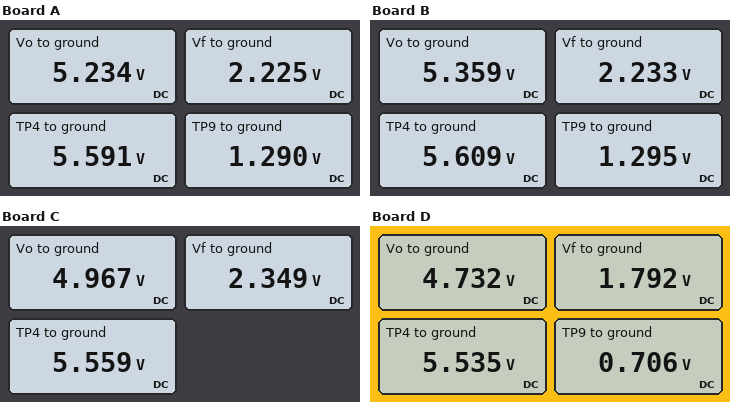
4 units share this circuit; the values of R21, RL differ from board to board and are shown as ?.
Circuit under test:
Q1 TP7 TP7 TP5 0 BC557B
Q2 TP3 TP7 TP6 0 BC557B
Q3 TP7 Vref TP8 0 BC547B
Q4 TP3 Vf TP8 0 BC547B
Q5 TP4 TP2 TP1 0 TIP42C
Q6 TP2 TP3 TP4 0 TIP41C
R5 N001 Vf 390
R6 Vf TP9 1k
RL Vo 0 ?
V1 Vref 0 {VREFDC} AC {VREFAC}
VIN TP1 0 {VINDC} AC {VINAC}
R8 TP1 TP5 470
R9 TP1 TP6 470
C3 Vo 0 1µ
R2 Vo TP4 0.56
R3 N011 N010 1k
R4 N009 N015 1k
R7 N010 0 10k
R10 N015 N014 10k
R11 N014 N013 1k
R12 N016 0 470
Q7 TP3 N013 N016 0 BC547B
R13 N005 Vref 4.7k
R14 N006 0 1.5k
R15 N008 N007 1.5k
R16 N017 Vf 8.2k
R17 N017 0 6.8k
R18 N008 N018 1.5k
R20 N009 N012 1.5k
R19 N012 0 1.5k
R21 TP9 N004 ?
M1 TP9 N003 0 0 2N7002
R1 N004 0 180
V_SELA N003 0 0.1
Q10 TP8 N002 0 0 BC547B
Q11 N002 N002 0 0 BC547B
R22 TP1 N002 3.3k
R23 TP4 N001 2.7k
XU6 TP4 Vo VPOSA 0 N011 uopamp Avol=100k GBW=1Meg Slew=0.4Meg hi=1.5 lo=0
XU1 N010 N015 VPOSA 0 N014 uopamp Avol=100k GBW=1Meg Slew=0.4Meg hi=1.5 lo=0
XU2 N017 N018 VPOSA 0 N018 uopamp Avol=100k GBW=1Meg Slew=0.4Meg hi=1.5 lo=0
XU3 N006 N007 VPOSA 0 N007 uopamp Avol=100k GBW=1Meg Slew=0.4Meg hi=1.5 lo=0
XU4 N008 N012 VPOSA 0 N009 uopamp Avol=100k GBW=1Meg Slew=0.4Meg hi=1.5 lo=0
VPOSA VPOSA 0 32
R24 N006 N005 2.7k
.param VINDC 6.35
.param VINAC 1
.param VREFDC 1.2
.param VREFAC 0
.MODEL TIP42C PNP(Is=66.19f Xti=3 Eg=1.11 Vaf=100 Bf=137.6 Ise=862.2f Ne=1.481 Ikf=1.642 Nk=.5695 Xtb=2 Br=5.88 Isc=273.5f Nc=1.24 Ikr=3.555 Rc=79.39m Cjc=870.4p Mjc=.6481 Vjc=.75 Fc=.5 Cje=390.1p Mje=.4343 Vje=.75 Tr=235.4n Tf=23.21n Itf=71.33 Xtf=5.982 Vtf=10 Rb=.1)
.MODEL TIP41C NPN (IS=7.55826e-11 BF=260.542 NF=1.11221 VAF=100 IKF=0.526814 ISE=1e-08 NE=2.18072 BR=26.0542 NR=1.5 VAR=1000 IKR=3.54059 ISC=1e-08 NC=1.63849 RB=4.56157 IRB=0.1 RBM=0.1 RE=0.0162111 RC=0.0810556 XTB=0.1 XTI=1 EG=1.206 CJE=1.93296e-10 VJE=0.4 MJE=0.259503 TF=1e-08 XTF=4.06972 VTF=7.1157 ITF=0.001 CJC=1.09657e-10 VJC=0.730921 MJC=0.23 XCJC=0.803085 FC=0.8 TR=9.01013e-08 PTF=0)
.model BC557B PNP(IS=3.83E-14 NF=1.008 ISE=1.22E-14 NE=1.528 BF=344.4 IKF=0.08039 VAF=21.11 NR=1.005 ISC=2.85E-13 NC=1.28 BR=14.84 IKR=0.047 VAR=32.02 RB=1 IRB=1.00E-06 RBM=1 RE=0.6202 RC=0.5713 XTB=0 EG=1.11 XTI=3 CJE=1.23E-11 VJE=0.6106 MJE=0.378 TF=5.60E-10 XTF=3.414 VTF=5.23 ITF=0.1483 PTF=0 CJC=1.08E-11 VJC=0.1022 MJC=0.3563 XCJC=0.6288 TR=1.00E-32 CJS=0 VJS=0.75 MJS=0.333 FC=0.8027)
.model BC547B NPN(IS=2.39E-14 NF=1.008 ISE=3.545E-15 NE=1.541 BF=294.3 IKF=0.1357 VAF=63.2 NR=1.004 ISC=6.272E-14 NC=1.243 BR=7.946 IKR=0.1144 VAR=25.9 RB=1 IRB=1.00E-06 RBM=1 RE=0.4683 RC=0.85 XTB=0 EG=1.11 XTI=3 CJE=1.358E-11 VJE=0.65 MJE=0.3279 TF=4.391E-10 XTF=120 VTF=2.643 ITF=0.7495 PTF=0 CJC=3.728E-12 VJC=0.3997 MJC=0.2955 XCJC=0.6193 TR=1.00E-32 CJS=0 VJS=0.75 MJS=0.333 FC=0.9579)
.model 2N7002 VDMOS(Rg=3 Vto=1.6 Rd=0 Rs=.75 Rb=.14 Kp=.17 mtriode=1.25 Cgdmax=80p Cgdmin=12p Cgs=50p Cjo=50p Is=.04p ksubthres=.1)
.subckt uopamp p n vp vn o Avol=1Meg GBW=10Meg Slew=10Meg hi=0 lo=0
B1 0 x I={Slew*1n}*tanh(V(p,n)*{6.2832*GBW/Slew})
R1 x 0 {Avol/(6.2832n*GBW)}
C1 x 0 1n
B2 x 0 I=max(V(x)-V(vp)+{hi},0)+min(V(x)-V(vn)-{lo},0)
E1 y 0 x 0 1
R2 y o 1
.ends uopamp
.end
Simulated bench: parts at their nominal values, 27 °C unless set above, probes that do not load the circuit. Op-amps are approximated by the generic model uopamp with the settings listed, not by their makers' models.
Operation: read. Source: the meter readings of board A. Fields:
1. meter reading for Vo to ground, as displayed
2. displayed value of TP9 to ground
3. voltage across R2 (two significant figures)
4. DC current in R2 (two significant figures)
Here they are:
5.234 V
1.290 V
360 mV
640 mA
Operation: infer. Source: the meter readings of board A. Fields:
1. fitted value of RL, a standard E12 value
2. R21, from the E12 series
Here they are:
8.2 Ω
1.2 kΩ
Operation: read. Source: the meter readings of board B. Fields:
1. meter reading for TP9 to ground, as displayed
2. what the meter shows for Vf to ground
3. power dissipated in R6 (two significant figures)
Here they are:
1.295 V
2.233 V
880 µW
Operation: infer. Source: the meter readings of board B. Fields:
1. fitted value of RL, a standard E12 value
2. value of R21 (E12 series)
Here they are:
12 Ω
1.2 kΩ
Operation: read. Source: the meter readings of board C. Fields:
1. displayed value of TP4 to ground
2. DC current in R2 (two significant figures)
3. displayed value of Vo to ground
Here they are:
5.559 V
1.1 A
4.967 V
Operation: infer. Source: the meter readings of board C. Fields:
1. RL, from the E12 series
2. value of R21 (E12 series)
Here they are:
4.7 Ω
1.5 kΩ
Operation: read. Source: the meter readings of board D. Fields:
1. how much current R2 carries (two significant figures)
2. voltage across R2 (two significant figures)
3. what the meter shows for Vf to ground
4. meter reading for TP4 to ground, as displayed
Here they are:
1.4 A
800 mV
1.792 V
5.535 V
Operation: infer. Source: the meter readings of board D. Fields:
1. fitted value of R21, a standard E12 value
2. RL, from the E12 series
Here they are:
470 Ω
3.3 Ω
